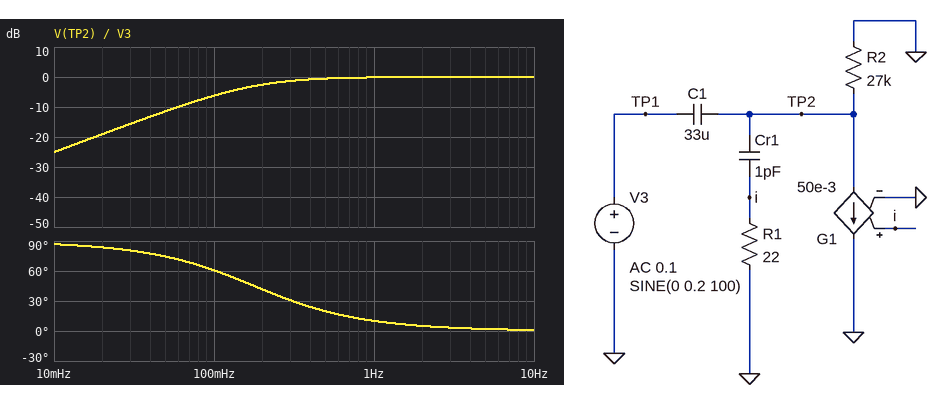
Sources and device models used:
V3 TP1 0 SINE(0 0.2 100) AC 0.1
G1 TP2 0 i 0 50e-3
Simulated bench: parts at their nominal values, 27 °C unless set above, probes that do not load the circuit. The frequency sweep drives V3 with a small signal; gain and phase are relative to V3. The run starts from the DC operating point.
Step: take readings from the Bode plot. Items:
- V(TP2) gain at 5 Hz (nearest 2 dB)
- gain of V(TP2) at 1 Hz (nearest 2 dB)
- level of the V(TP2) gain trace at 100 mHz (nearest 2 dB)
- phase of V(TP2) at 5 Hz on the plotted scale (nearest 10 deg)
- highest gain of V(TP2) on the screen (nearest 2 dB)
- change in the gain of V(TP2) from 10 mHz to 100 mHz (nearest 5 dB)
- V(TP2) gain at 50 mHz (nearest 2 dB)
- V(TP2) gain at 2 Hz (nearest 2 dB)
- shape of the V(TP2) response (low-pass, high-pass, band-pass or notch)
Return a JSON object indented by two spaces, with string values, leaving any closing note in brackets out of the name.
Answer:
{
  "V(TP2) gain at 5 Hz": "0 dB",
  "gain of V(TP2) at 1 Hz": "0 dB",
  "level of the V(TP2) gain trace at 100 mHz": "-6 dB",
  "phase of V(TP2) at 5 Hz on the plotted scale": "0 deg",
  "highest gain of V(TP2) on the screen": "0 dB",
  "change in the gain of V(TP2) from 10 mHz to 100 mHz": "20 dB",
  "V(TP2) gain at 50 mHz": "-12 dB",
  "V(TP2) gain at 2 Hz": "0 dB",
  "shape of the V(TP2) response": "high-pass"
}
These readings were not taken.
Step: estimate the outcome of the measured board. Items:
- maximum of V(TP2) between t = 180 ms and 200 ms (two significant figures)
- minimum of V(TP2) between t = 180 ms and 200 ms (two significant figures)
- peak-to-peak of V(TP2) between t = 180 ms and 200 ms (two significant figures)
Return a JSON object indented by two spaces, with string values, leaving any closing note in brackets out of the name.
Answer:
{
  "maximum of V(TP2) between t = 180 ms and 200 ms": "200 mV",
  "minimum of V(TP2) between t = 180 ms and 200 ms": "-200 mV",
  "peak-to-peak of V(TP2) between t = 180 ms and 200 ms": "400 mV"
}
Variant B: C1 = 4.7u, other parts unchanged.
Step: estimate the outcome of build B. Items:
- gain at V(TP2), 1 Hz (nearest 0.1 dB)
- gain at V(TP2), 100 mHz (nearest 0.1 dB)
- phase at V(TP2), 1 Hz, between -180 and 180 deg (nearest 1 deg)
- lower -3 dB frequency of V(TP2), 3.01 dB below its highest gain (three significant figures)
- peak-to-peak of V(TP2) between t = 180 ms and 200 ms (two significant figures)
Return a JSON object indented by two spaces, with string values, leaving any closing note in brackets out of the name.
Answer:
{
  "gain at V(TP2), 1 Hz": "-4.1 dB",
  "gain at V(TP2), 100 mHz": "-22.0 dB",
  "phase at V(TP2), 1 Hz, between -180 and 180 deg": "51 deg",
  "lower -3 dB frequency of V(TP2), 3.01 dB below its highest gain": "1.25 Hz",
  "peak-to-peak of V(TP2) between t = 180 ms and 200 ms": "400 mV"
}
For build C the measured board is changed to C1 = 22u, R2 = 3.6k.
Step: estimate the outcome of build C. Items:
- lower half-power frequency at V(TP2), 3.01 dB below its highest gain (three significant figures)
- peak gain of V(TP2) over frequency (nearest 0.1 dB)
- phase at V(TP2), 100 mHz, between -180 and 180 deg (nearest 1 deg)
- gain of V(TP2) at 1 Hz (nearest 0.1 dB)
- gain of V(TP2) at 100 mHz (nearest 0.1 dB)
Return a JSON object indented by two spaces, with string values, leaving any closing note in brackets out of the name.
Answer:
{
  "lower half-power frequency at V(TP2), 3.01 dB below its highest gain": "2.01 Hz",
  "peak gain of V(TP2) over frequency": "0 dB",
  "phase at V(TP2), 100 mHz, between -180 and 180 deg": "87 deg",
  "gain of V(TP2) at 1 Hz": "-7.0 dB",
  "gain of V(TP2) at 100 mHz": "-26.1 dB"
}
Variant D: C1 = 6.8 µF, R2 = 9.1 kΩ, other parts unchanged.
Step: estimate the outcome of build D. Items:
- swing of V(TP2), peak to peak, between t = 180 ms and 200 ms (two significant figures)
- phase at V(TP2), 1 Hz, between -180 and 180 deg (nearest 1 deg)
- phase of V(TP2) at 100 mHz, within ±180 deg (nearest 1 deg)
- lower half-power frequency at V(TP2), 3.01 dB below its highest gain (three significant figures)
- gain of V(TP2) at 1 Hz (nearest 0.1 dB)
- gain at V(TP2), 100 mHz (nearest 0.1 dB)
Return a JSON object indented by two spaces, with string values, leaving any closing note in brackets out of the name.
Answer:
{
  "swing of V(TP2), peak to peak, between t = 180 ms and 200 ms": "400 mV",
  "phase at V(TP2), 1 Hz, between -180 and 180 deg": "69 deg",
  "phase of V(TP2) at 100 mHz, within ±180 deg": "88 deg",
  "lower half-power frequency at V(TP2), 3.01 dB below its highest gain": "2.57 Hz",
  "gain of V(TP2) at 1 Hz": "-8.8 dB",
  "gain at V(TP2), 100 mHz": "-28.2 dB"
}
